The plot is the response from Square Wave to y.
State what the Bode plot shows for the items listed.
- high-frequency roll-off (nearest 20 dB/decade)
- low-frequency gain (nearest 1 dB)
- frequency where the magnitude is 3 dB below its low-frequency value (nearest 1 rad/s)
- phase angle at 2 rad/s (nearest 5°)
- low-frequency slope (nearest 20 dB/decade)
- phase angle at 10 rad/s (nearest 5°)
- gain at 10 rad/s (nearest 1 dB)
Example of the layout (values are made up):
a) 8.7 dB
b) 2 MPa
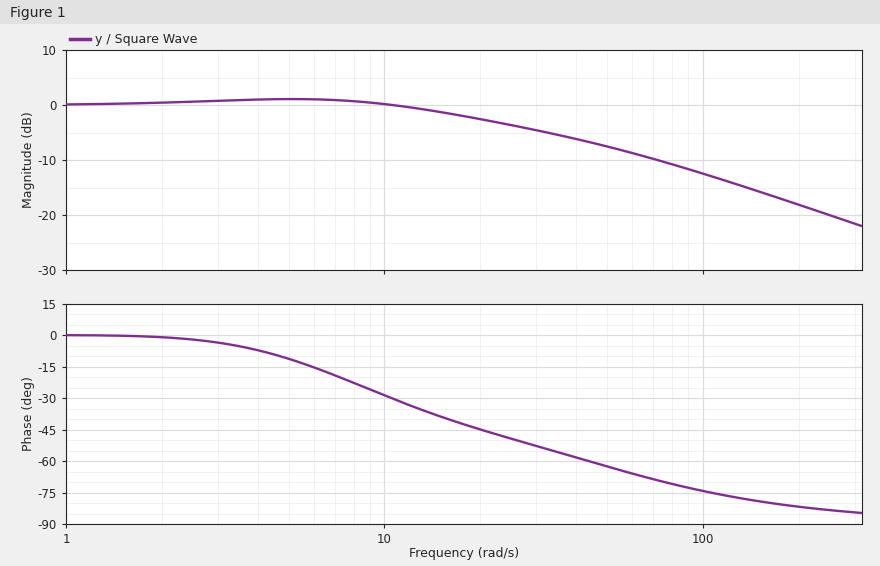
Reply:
a) -20 dB/decade
b) 0 dB
c) 21 rad/s
d) 0°
e) 0 dB/decade
f) -30°
g) 0 dB
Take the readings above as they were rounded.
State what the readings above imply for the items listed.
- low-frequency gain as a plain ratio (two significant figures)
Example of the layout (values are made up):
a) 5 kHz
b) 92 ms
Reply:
a) 1.0
